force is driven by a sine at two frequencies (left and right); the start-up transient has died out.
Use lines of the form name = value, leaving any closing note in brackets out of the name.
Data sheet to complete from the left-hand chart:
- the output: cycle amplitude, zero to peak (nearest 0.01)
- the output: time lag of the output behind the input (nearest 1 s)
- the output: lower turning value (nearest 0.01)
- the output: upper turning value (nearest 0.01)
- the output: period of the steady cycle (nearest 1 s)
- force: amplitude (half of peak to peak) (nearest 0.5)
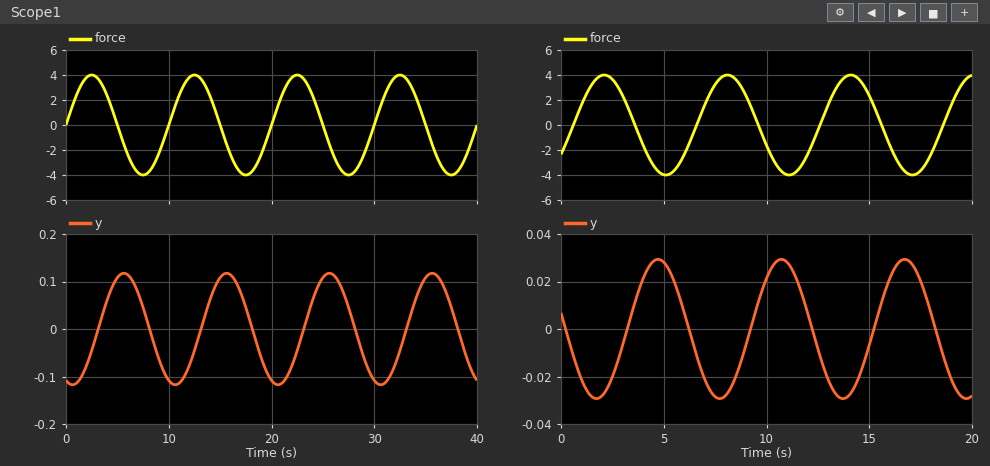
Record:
the output: cycle amplitude, zero to peak = 0.12
the output: time lag of the output behind the input = 3 s
the output: lower turning value = -0.12
the output: upper turning value = 0.12
the output: period of the steady cycle = 10 s
force: amplitude (half of peak to peak) = 4.0
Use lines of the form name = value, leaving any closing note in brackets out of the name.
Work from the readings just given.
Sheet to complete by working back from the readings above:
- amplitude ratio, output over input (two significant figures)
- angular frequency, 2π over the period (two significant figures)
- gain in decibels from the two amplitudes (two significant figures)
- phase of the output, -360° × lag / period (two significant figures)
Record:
amplitude ratio, output over input = 0.030
angular frequency, 2π over the period = 0.63 rad/s
gain in decibels from the two amplitudes = -30 dB
phase of the output, -360° × lag / period = -110°
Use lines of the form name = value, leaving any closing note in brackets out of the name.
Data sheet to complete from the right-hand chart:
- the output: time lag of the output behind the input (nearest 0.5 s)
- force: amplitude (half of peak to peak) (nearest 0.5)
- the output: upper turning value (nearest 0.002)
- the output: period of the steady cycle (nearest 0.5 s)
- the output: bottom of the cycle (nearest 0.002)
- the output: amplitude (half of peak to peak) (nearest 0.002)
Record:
the output: time lag of the output behind the input = 2.5 s
force: amplitude (half of peak to peak) = 4.0
the output: upper turning value = 0.030
the output: period of the steady cycle = 6.0 s
the output: bottom of the cycle = -0.030
the output: amplitude (half of peak to peak) = 0.030
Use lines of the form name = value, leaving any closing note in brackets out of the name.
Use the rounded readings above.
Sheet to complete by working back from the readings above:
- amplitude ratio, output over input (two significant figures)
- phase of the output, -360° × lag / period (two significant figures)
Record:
amplitude ratio, output over input = 0.0075
phase of the output, -360° × lag / period = -150°
